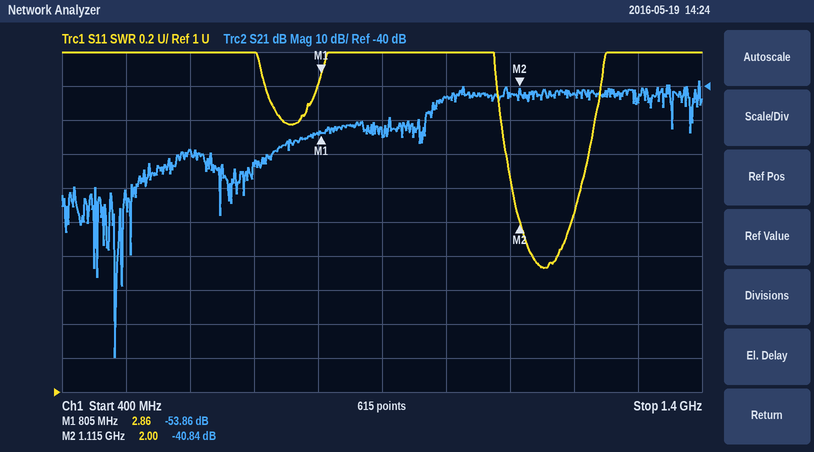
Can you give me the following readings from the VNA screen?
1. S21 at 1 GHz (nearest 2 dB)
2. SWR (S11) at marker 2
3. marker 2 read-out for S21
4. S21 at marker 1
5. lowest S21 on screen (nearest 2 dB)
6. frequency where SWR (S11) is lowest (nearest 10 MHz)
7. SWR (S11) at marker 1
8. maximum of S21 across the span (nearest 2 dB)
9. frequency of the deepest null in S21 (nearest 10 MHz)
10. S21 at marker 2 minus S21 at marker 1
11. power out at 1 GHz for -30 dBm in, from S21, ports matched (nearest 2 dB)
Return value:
-44 dB
2.00
-40.84 dB
-53.86 dB
-120 dB
1.15 GHz
2.86
-38 dB
480 MHz
13.02 dB
-74 dBm
